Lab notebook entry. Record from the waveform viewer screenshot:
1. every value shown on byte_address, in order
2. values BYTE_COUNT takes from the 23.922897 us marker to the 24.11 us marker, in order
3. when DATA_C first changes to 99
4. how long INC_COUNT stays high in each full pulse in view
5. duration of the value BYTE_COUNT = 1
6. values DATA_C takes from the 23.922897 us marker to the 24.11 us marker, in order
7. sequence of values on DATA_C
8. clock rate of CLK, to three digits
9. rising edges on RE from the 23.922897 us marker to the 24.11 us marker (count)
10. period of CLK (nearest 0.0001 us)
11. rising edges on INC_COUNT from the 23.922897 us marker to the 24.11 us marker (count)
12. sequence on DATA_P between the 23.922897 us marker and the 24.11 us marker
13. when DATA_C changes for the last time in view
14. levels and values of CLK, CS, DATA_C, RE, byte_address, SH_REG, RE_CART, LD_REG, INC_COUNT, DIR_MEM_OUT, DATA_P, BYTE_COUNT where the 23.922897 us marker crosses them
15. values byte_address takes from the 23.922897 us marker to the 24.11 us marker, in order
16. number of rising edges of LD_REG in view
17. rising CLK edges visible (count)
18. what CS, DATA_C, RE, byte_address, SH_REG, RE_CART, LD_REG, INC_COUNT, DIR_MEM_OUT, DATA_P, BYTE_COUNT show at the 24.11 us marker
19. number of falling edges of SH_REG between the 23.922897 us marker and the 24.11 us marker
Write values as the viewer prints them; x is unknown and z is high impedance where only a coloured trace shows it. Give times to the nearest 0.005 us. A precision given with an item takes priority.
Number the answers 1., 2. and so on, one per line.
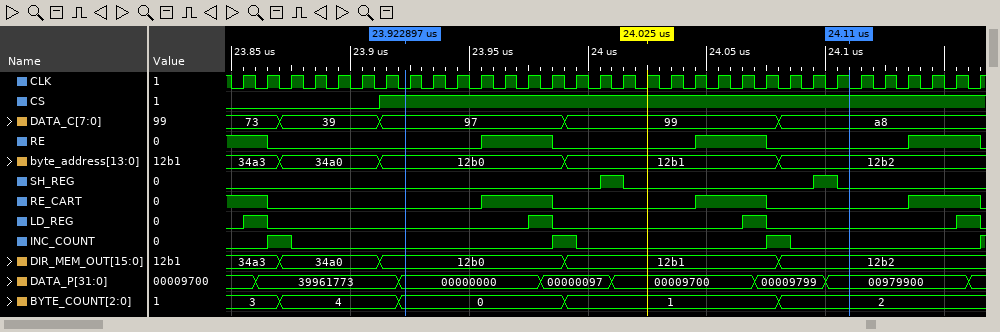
1. 34a3, 34a0, 12b0, 12b1, 12b2
2. 0, 1, 2
3. 23.99 us
4. 0.01 us, 0.01 us, 0.01 us
5. 0.09 us
6. 97, 99, a8
7. 73, 39, 97, 99, a8
8. 100 MHz
9. 2
10. 0.01 us
11. 2
12. 00000000, 00000097, 00009700, 00009799, 00979900
13. 24.08 us
14. CLK=0, CS=1, DATA_C=97, RE=0, byte_address=12b0, SH_REG=0, RE_CART=0, LD_REG=0, INC_COUNT=0, DIR_MEM_OUT=12b0, DATA_P=00000000, BYTE_COUNT=0
15. 12b0, 12b1, 12b2
16. 4
17. 32
18. CS=1, DATA_C=a8, RE=0, byte_address=12b2, SH_REG=0, RE_CART=0, LD_REG=0, INC_COUNT=0, DIR_MEM_OUT=12b2, DATA_P=00979900, BYTE_COUNT=2
19. 2
